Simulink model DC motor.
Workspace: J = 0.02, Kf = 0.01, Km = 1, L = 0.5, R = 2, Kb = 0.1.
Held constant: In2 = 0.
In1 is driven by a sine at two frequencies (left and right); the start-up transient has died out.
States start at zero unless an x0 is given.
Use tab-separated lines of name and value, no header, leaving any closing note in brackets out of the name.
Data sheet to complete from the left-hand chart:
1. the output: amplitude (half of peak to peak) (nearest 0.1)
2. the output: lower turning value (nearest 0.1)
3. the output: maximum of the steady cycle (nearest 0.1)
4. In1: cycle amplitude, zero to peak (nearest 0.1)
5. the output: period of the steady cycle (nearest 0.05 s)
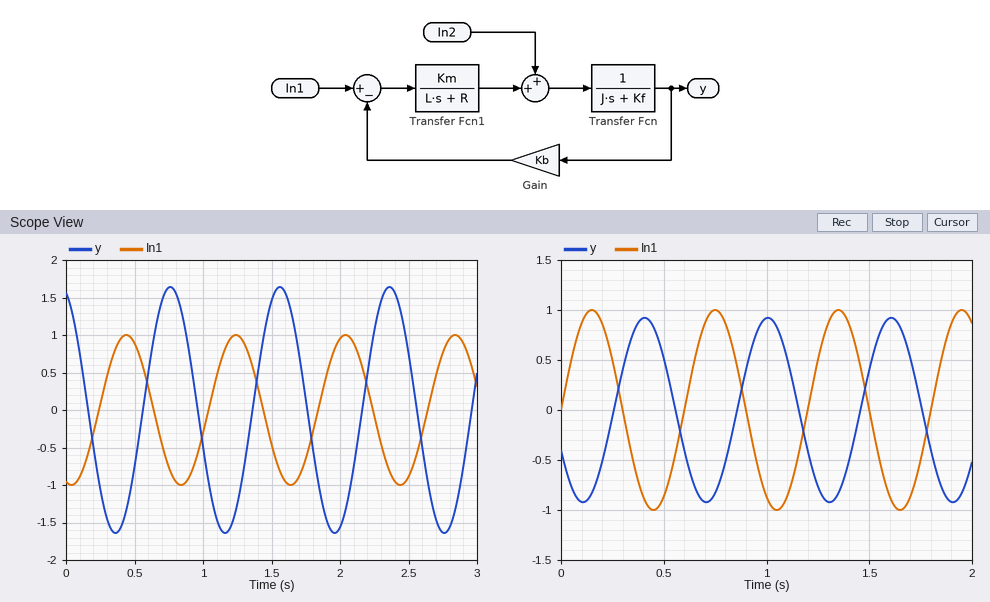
the output: amplitude (half of peak to peak)	1.6
the output: lower turning value	-1.6
the output: maximum of the steady cycle	1.6
In1: cycle amplitude, zero to peak	1.0
the output: period of the steady cycle	0.80 s
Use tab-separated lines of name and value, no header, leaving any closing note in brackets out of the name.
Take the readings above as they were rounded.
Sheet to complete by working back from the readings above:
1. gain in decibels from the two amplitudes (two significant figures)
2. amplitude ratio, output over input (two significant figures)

gain in decibels from the two amplitudes	4.1 dB
amplitude ratio, output over input	1.6
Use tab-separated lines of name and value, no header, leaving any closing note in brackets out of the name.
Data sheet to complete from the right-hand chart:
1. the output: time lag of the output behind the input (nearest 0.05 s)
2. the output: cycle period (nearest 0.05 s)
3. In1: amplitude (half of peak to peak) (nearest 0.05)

the output: time lag of the output behind the input	0.25 s
the output: cycle period	0.60 s
In1: amplitude (half of peak to peak)	1.00
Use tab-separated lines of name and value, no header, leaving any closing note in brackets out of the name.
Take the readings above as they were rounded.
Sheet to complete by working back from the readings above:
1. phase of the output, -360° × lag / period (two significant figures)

phase of the output, -360° × lag / period	-150°
